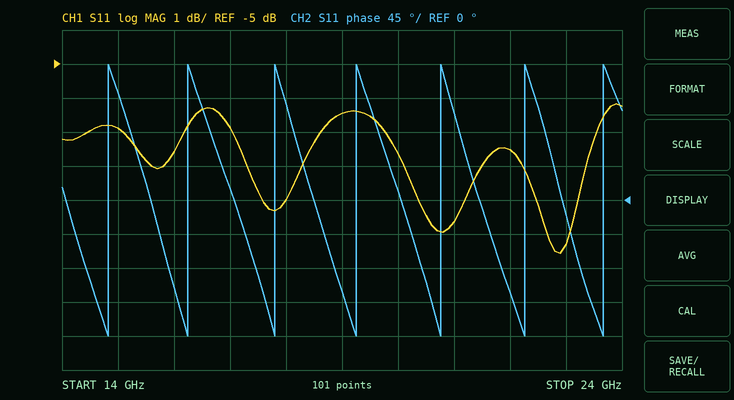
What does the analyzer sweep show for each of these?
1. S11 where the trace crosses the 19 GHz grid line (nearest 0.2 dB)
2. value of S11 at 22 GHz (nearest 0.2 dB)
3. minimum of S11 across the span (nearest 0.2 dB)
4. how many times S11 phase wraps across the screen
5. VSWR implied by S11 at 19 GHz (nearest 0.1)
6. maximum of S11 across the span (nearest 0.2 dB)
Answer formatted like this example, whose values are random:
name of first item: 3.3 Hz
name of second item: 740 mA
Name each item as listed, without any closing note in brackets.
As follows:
S11 where the trace crosses the 19 GHz grid line: -6.4 dB
value of S11 at 22 GHz: -7.6 dB
minimum of S11 across the span: -10.6 dB
how many times S11 phase wraps across the screen: 7
VSWR implied by S11 at 19 GHz: 2.8
maximum of S11 across the span: -6.2 dB
